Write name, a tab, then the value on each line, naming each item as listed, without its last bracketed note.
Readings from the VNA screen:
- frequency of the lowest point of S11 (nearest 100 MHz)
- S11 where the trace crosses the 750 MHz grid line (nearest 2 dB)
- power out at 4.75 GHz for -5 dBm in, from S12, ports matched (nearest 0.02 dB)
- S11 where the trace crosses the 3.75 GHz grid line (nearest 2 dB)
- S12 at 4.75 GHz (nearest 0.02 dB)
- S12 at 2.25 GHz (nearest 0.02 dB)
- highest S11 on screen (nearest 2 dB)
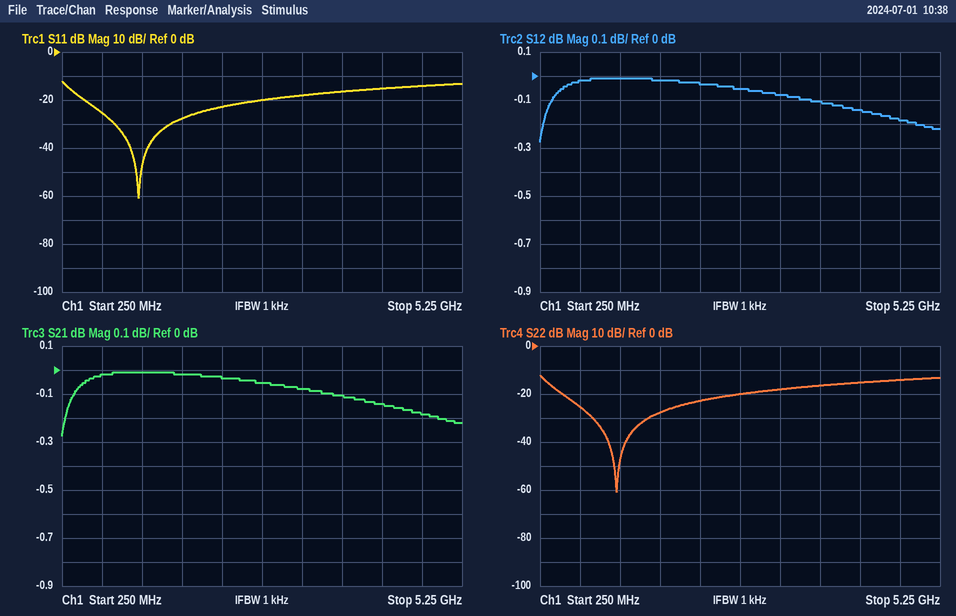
frequency of the lowest point of S11	1.2 GHz
S11 where the trace crosses the 750 MHz grid line	-26 dB
power out at 4.75 GHz for -5 dBm in, from S12, ports matched	-5.18 dBm
S11 where the trace crosses the 3.75 GHz grid line	-16 dB
S12 at 4.75 GHz	-0.18 dB
S12 at 2.25 GHz	-0.04 dB
highest S11 on screen	-12 dB
